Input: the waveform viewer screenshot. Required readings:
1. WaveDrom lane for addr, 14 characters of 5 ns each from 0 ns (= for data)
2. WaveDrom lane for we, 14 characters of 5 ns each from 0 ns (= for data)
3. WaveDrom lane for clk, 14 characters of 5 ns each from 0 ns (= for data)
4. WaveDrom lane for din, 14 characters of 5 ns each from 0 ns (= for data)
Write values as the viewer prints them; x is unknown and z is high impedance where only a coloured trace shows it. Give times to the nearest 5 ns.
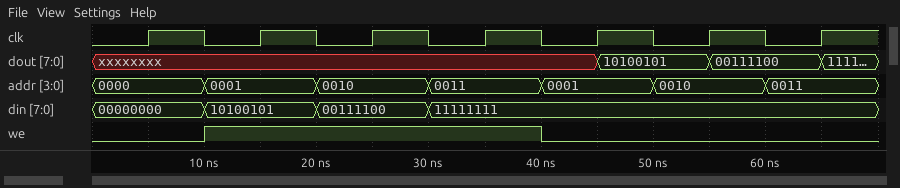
{name: 'addr', wave: '=.=.=.=.=.=.=.', data: '0000 0001 0010 0011 0001 0010 0011'}
{name: 'we', wave: '0.1.....0.....'}
{name: 'clk', wave: '01010101010101'}
{name: 'din', wave: '=.=.=.=.......', data: '00000000 10100101 00111100 11111111'}
